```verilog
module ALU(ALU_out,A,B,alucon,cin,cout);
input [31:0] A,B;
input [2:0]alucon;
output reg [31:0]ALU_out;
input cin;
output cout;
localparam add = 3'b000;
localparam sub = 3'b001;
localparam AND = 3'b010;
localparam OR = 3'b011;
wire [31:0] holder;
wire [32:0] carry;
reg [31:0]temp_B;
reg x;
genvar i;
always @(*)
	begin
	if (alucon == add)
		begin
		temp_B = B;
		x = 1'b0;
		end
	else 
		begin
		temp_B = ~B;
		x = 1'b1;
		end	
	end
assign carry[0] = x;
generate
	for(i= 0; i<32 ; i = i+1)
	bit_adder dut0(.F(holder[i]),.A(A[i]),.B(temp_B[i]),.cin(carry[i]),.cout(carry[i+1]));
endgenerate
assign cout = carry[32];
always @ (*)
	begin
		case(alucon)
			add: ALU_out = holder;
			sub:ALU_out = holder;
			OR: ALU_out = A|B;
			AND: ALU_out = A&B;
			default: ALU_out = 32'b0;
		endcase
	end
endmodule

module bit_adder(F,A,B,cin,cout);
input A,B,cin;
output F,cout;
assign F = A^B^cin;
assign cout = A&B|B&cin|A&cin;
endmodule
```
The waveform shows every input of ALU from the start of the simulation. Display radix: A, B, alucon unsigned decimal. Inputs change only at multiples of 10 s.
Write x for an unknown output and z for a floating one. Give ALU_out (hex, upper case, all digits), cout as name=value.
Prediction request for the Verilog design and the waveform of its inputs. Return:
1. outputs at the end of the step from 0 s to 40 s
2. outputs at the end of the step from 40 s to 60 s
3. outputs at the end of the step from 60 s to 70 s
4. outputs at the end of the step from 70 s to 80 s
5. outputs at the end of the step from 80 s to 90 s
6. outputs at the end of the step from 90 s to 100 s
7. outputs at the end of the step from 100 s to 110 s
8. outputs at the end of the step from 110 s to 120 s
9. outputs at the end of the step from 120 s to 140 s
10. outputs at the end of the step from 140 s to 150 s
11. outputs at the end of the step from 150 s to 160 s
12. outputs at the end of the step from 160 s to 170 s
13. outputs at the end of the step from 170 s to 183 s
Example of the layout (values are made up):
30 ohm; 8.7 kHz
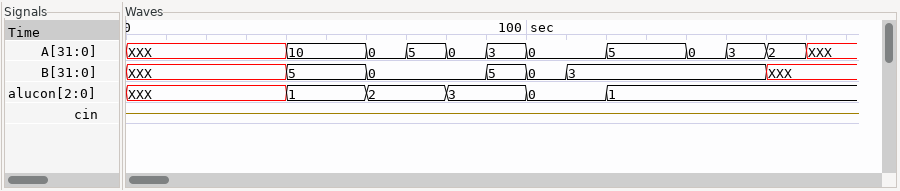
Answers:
ALU_out=x, cout=x; ALU_out=00000005, cout=1; ALU_out=00000000, cout=1; ALU_out=00000000, cout=1; ALU_out=00000000, cout=1; ALU_out=00000007, cout=0; ALU_out=00000000, cout=0; ALU_out=00000003, cout=0; ALU_out=00000002, cout=1; ALU_out=FFFFFFFD, cout=0; ALU_out=00000000, cout=1; ALU_out=x, cout=x; ALU_out=x, cout=x
